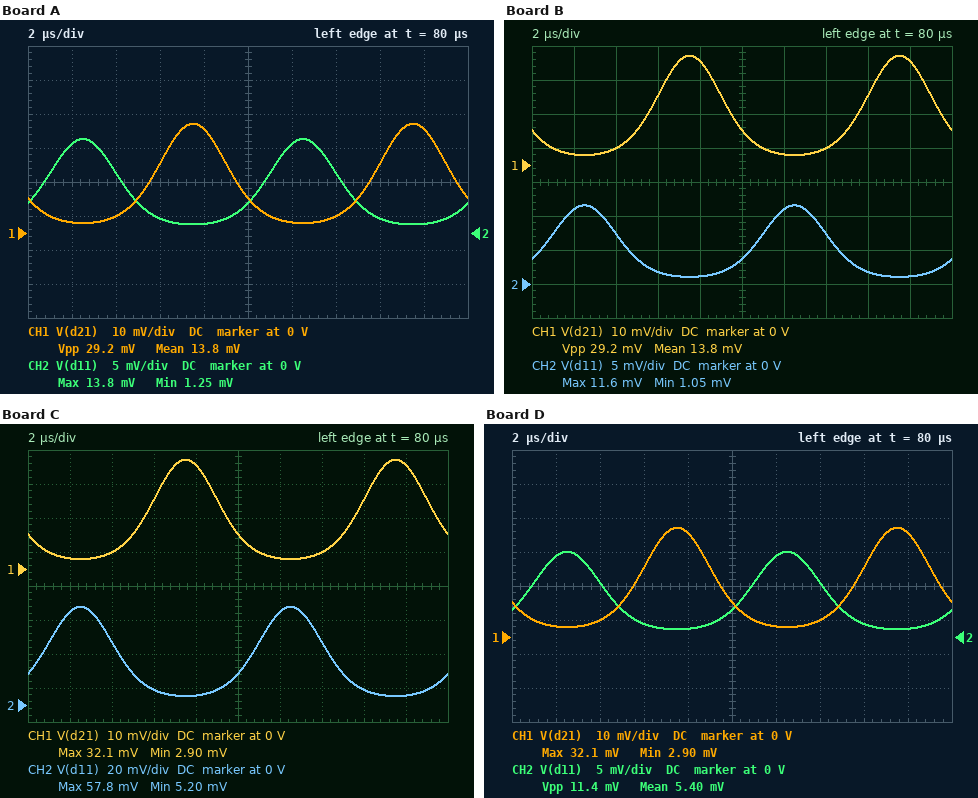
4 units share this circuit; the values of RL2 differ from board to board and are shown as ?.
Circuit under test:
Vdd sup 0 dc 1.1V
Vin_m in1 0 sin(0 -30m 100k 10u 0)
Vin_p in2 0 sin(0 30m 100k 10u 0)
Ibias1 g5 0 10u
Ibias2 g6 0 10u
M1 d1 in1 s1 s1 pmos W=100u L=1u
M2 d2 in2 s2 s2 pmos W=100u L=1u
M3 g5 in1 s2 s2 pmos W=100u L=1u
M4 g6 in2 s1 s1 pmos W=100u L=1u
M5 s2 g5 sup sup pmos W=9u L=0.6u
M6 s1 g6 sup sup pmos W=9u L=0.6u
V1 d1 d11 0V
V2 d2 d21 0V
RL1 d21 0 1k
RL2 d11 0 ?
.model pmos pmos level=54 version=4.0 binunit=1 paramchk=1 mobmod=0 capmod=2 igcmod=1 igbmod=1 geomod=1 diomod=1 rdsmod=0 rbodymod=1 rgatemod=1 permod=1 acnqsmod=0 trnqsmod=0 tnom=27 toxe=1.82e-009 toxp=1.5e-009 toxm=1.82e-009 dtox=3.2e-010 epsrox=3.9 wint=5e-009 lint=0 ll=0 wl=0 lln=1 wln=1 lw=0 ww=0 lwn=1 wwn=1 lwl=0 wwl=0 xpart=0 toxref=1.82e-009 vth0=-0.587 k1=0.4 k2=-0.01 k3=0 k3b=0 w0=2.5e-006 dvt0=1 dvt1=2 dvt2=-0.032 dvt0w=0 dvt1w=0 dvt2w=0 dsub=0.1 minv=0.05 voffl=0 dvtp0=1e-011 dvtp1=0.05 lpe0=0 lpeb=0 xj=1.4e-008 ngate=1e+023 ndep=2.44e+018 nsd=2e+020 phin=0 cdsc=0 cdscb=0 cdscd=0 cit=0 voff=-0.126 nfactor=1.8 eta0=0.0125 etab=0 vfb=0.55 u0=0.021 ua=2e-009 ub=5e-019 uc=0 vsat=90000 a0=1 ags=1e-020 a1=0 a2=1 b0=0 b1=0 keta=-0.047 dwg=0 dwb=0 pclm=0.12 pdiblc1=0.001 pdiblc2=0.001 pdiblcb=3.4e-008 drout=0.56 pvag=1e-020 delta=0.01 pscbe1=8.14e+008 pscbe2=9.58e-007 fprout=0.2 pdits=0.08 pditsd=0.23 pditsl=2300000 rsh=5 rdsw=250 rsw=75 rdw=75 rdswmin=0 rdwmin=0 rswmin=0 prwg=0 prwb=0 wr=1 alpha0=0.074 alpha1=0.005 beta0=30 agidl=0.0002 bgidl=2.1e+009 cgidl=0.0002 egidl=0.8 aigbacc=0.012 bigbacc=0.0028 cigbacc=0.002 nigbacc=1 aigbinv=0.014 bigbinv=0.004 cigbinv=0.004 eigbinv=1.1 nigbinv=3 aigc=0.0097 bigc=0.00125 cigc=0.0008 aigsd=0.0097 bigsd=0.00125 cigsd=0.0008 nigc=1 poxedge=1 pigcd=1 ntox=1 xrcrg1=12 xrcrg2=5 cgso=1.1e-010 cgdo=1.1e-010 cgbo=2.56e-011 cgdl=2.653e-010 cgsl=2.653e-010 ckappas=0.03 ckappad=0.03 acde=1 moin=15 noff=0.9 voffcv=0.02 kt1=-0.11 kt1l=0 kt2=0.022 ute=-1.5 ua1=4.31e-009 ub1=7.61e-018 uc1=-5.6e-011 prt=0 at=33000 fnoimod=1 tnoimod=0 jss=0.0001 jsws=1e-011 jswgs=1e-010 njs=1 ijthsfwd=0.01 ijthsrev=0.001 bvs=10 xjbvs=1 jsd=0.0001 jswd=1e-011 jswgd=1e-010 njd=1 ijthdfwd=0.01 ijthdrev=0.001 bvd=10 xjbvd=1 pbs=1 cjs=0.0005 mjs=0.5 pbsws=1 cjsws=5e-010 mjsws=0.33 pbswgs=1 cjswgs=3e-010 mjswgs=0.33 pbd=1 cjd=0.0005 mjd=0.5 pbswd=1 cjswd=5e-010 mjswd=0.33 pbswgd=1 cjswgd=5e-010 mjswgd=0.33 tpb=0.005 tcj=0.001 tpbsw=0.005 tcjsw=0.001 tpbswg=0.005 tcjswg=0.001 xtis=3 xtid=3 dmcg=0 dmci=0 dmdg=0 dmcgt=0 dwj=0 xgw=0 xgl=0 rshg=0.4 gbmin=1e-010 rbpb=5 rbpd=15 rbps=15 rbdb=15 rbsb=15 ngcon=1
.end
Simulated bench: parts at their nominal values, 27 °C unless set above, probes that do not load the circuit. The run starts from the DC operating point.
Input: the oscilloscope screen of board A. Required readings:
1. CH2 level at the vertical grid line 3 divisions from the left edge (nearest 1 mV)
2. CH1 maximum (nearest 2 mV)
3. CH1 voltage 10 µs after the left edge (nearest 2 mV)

2 mV
32 mV
10 mV
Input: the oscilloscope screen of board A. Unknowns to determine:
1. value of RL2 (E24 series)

430 Ω
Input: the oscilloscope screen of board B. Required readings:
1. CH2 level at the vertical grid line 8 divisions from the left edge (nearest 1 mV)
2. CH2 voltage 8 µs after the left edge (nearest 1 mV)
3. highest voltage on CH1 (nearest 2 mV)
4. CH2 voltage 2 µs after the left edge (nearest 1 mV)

2 mV
1 mV
32 mV
11 mV
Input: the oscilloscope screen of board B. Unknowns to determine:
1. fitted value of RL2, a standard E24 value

360 Ω
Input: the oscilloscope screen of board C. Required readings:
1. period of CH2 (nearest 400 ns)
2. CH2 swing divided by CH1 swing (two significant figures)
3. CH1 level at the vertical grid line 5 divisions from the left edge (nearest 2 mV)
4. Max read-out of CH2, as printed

10.0 µs
1.8
10 mV
57.8 mV
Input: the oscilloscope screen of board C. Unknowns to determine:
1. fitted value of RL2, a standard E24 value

1.8 kΩ
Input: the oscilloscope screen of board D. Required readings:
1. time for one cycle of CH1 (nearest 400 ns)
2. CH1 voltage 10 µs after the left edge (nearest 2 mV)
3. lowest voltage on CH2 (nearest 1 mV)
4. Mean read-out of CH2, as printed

10.0 µs
10 mV
1 mV
5.40 mV
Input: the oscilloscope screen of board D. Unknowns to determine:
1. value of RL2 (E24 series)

390 Ω
